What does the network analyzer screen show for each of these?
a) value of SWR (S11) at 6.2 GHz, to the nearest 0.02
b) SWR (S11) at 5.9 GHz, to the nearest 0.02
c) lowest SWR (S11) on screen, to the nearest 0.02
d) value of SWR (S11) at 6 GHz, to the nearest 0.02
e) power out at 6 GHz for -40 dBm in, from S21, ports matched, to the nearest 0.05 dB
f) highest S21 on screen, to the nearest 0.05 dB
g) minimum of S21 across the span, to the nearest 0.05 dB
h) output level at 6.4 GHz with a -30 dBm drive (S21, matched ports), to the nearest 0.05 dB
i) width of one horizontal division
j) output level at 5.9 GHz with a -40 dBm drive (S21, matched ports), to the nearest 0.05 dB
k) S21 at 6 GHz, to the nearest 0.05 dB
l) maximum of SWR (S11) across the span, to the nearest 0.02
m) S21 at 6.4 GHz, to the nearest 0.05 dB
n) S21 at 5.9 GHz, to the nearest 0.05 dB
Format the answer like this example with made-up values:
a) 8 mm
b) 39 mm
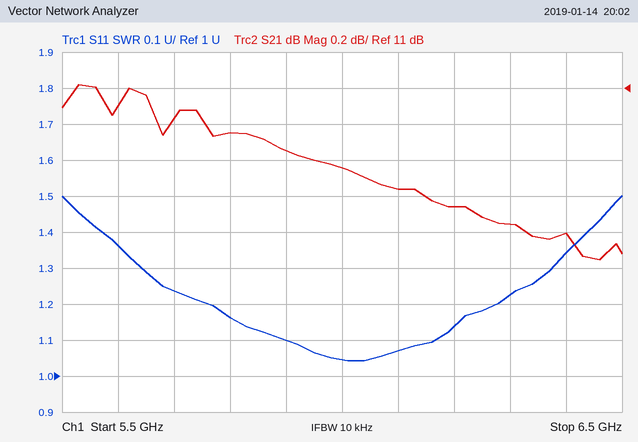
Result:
a) 1.14
b) 1.10
c) 1.04
d) 1.04
e) -29.45 dBm
f) 11.00 dB
g) 10.05 dB
h) -19.80 dBm
i) 100 MHz
j) -29.35 dBm
k) 10.55 dB
l) 1.50
m) 10.20 dB
n) 10.65 dB
